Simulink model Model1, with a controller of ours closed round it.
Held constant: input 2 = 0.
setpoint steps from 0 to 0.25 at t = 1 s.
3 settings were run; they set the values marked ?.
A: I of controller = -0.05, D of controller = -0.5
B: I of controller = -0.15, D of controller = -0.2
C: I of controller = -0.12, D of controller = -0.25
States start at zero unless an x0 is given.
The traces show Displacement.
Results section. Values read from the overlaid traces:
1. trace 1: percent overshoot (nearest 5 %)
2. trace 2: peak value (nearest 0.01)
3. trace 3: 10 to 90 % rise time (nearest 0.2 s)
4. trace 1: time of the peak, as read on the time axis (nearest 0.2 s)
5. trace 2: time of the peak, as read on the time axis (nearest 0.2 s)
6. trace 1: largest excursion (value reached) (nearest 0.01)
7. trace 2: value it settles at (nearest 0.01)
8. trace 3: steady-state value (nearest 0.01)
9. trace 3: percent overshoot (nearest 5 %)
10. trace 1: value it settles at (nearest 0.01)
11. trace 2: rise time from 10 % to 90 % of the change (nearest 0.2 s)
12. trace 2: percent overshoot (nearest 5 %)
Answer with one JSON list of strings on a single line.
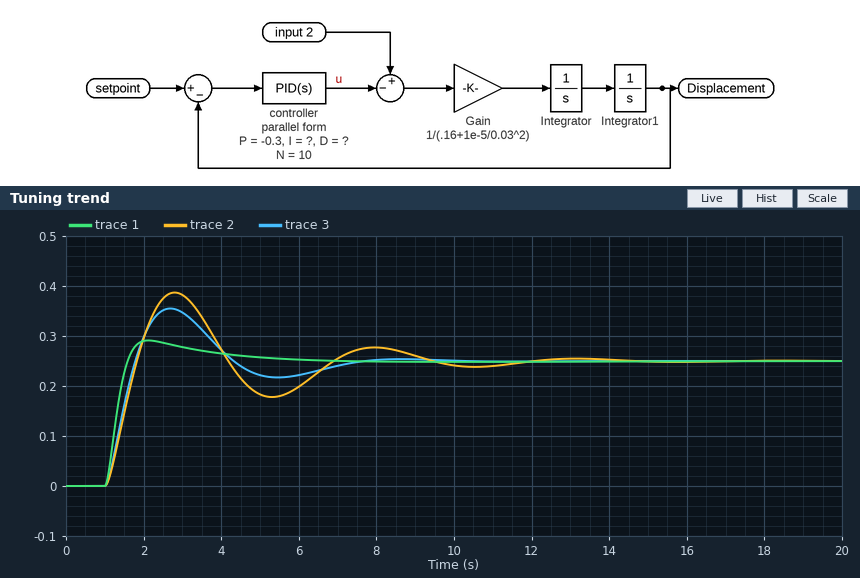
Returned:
["15 %", "0.39", "0.6 s", "2.2 s", "2.8 s", "0.29", "0.25", "0.25", "40 %", "0.25", "0.6 s", "55 %"]
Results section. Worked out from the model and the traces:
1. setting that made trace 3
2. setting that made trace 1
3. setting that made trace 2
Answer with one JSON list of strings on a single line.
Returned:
["C", "A", "B"]
